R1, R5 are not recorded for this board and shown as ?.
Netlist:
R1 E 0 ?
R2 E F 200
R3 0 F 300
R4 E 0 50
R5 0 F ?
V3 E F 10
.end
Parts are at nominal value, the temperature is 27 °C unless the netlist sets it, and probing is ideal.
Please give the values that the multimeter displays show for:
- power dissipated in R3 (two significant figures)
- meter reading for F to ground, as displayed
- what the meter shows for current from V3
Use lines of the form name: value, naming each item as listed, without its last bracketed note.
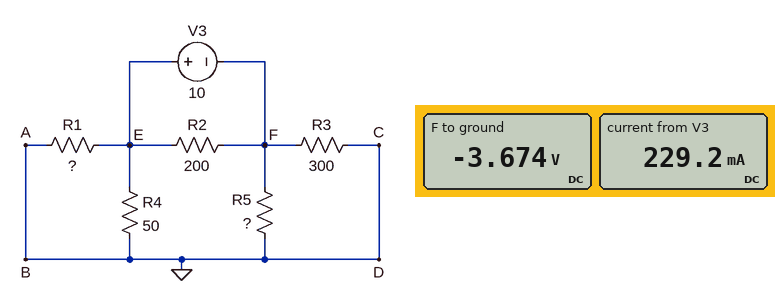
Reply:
power dissipated in R3: 45 mW
meter reading for F to ground, as displayed: -3.674 V
what the meter shows for current from V3: 229.2 mA
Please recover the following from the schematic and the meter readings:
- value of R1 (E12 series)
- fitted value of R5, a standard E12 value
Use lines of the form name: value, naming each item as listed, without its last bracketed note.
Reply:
value of R1: 120 Ω
fitted value of R5, a standard E12 value: 22 Ω
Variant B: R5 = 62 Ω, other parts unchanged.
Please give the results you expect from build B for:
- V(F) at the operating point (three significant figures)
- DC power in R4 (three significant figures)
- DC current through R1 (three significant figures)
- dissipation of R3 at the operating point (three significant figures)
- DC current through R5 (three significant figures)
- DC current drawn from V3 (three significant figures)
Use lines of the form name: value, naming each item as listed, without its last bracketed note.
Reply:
V(F) at the operating point: -5.93 V
DC power in R4: 332 mW
DC current through R1: 33.9 mA
dissipation of R3 at the operating point: 117 mW
DC current through R5: 95.6 mA
DC current drawn from V3: 165 mA
